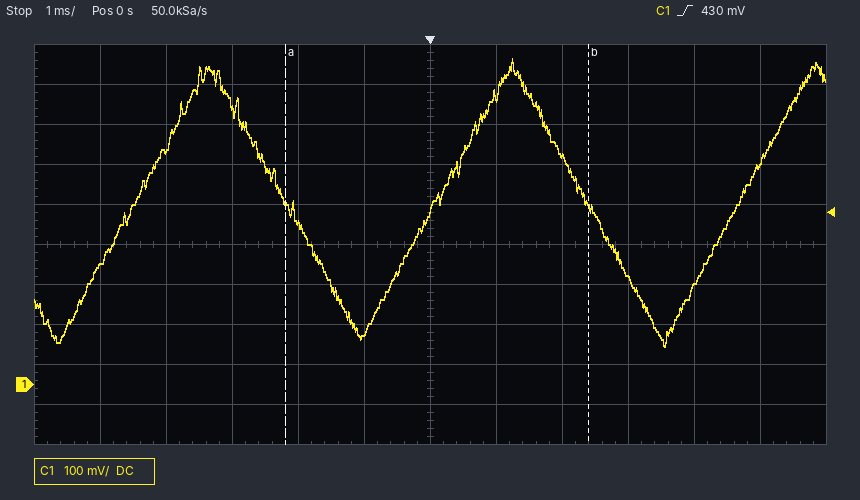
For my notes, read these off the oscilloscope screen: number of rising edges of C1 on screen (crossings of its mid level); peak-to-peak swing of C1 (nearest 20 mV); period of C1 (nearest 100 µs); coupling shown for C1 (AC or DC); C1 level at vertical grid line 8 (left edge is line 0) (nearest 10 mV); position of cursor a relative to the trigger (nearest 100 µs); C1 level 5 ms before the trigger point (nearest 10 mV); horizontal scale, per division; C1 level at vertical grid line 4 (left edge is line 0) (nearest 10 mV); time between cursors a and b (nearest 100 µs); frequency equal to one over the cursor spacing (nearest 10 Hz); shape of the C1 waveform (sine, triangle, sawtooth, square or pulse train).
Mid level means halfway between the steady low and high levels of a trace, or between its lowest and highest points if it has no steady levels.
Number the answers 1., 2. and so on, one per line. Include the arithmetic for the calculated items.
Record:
1. 3
2. 720 mV
3. 4.6 ms
4. DC
5. 570 mV
6. -2.2 ms
7. 300 mV
8. 1 ms
9. 400 mV
10. 4.6 ms
11. 1 / 4.6 ms ≈ 220 Hz
12. triangle
